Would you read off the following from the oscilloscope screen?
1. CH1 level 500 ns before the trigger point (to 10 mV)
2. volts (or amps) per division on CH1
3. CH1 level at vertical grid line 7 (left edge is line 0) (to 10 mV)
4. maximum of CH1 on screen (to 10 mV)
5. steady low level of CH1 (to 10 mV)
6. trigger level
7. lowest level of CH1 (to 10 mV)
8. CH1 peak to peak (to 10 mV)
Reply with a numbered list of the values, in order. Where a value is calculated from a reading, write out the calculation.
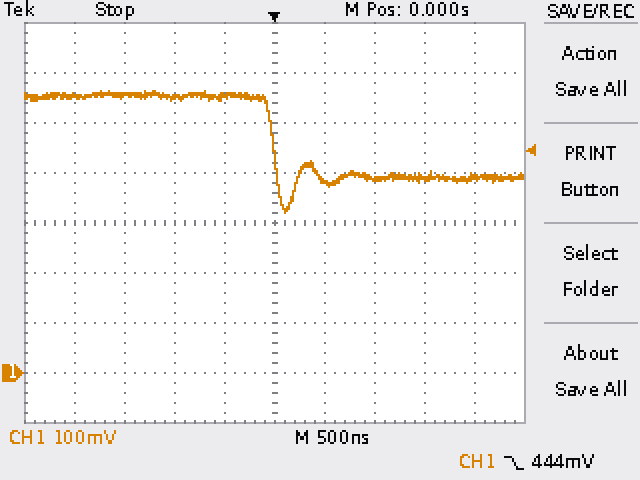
1. 550 mV
2. 100 mV
3. 390 mV
4. 560 mV
5. 390 mV
6. 444 mV
7. 320 mV
8. 560 mV − (320 mV) = 240 mV
